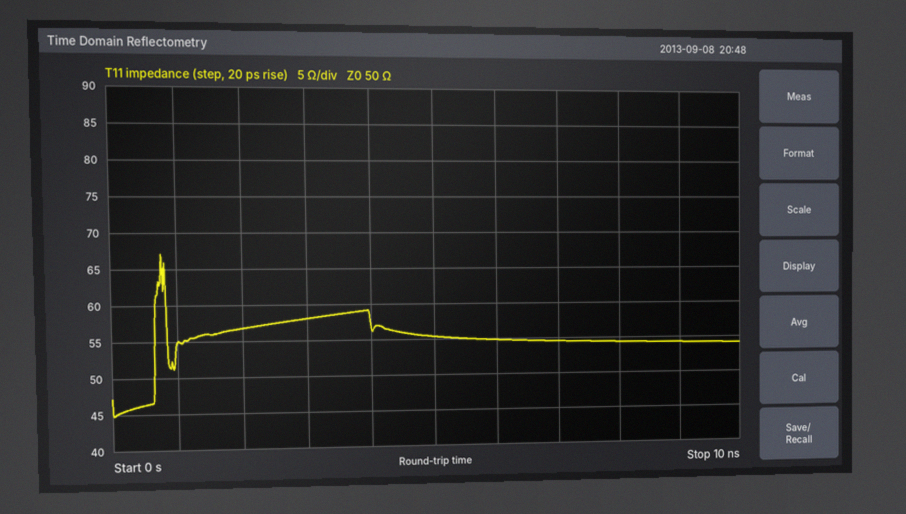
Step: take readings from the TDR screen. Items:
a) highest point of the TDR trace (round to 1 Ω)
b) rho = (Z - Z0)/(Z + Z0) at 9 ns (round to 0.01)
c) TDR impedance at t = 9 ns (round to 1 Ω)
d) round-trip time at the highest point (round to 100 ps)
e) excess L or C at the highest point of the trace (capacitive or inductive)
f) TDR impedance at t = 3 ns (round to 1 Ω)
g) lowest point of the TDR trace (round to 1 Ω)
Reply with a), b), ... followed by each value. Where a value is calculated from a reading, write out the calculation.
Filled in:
a) 67 Ω
b) (54 − 50)/(54 + 50) ≈ +0.04
c) 54 Ω
d) 800 ps
e) inductive
f) 58 Ω
g) 45 Ω
